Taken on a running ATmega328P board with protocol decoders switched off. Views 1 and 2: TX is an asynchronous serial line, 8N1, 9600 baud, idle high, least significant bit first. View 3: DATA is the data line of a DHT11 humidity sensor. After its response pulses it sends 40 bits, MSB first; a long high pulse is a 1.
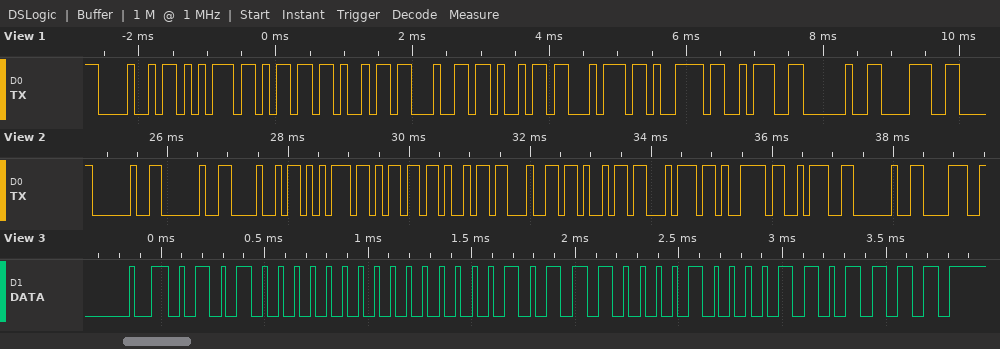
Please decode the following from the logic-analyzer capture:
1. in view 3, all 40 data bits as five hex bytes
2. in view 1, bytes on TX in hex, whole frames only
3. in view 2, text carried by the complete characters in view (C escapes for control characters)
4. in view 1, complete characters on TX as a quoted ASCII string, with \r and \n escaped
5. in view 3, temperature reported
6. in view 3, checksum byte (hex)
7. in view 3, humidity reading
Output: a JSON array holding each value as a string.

["50 00 17 08 6F", "48 75 6D 69 64 69 74 79 3A 20 38", "\"  Humidity: 8\"", "\"Humidity: 8\"", "23.8 °C", "0x6F", "80 %"]
